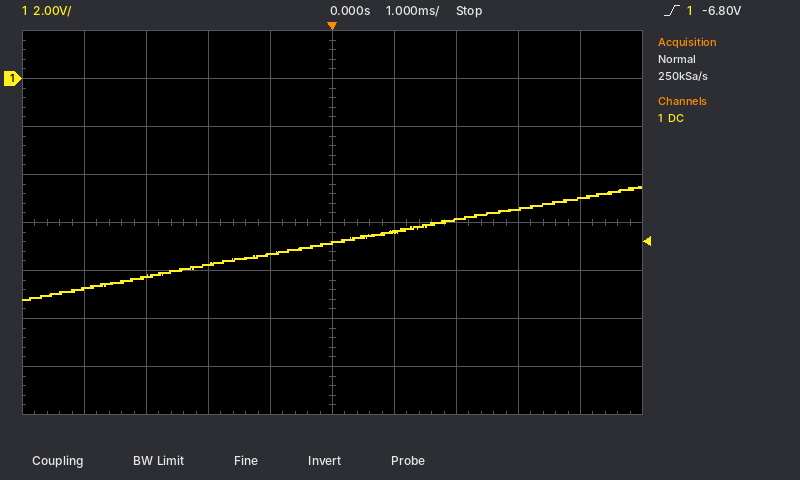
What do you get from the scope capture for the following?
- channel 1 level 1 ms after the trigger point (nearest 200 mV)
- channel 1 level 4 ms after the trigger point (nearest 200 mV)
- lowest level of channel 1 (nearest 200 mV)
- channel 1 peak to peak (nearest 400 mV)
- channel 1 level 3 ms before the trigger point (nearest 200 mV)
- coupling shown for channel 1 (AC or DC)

-6.4 V
-5.0 V
-9.2 V
4.8 V
-8.2 V
DC
